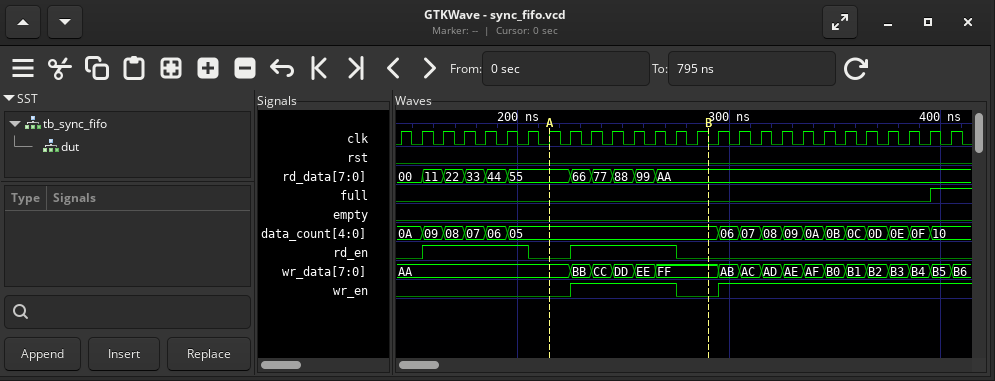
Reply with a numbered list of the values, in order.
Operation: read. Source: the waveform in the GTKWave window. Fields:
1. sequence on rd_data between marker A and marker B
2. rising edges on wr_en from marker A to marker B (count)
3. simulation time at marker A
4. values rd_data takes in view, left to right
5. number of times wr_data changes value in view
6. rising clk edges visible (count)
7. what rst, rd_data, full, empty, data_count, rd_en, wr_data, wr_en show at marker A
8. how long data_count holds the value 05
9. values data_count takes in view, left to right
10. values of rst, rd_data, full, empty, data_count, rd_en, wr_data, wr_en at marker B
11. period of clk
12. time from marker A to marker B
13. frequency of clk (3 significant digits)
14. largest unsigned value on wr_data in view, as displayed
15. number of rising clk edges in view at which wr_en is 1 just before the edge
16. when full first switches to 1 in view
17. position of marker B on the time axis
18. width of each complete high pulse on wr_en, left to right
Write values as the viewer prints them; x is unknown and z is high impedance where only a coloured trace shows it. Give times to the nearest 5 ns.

1. 55, 66, 77, 88, 99, AA
2. 1
3. 215 ns
4. 00, 11, 22, 33, 44, 55, 66, 77, 88, 99, AA
5. 17
6. 27
7. rst=0, rd_data=55, full=0, empty=0, data_count=05, rd_en=0, wr_data=AA, wr_en=0
8. 100 ns
9. 0A, 09, 08, 07, 06, 05, 06, 07, 08, 09, 0A, 0B, 0C, 0D, 0E, 0F, 10
10. rst=0, rd_data=AA, full=0, empty=0, data_count=05, rd_en=0, wr_data=FF, wr_en=0
11. 10 ns
12. 75 ns
13. 100 MHz
14. FF
15. 16
16. 395 ns
17. 290 ns
18. 50 ns
